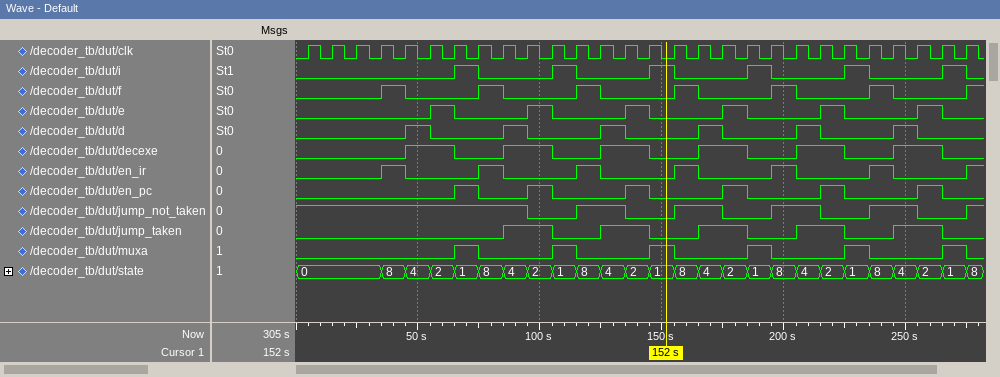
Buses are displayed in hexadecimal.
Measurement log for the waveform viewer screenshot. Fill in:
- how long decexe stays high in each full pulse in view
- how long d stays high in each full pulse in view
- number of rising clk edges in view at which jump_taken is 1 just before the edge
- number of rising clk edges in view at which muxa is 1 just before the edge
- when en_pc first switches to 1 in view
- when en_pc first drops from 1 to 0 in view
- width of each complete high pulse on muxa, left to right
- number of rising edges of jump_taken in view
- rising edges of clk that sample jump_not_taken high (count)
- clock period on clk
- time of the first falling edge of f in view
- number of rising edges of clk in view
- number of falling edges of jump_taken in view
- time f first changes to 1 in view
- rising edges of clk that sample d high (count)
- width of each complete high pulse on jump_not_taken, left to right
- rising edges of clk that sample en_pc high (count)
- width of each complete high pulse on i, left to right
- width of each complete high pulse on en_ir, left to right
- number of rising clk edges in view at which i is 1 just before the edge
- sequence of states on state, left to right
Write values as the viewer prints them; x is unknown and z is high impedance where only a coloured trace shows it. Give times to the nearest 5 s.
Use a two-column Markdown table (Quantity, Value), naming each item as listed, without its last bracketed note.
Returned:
| Quantity | Value |
|---|---|
| how long decexe stays high in each full pulse in view | 20 s, 20 s, 20 s, 20 s, 20 s, 20 s |
| how long d stays high in each full pulse in view | 10 s, 10 s, 10 s, 10 s, 10 s, 10 s |
| number of rising clk edges in view at which jump_taken is 1 just before the edge | 10 |
| number of rising clk edges in view at which muxa is 1 just before the edge | 6 |
| when en_pc first switches to 1 in view | 65 s |
| when en_pc first drops from 1 to 0 in view | 75 s |
| width of each complete high pulse on muxa, left to right | 10 s, 10 s, 10 s, 10 s, 10 s, 10 s |
| number of rising edges of jump_taken in view | 5 |
| rising edges of clk that sample jump_not_taken high | 18 |
| clock period on clk | 10 s |
| time of the first falling edge of f in view | 45 s |
| number of rising edges of clk in view | 28 |
| number of falling edges of jump_taken in view | 5 |
| time f first changes to 1 in view | 35 s |
| rising edges of clk that sample d high | 6 |
| width of each complete high pulse on jump_not_taken, left to right | 20 s, 20 s, 20 s, 20 s |
| rising edges of clk that sample en_pc high | 6 |
| width of each complete high pulse on i, left to right | 10 s, 10 s, 10 s, 10 s, 10 s, 10 s |
| width of each complete high pulse on en_ir, left to right | 10 s, 10 s, 10 s, 10 s, 10 s, 10 s |
| number of rising clk edges in view at which i is 1 just before the edge | 6 |
| sequence of states on state, left to right | 0, 8, 4, 2, 1, 8, 4, 2, 1, 8, 4, 2, 1, 8, 4, 2, 1, 8, 4, 2, 1, 8, 4, 2, 1, 8 |
